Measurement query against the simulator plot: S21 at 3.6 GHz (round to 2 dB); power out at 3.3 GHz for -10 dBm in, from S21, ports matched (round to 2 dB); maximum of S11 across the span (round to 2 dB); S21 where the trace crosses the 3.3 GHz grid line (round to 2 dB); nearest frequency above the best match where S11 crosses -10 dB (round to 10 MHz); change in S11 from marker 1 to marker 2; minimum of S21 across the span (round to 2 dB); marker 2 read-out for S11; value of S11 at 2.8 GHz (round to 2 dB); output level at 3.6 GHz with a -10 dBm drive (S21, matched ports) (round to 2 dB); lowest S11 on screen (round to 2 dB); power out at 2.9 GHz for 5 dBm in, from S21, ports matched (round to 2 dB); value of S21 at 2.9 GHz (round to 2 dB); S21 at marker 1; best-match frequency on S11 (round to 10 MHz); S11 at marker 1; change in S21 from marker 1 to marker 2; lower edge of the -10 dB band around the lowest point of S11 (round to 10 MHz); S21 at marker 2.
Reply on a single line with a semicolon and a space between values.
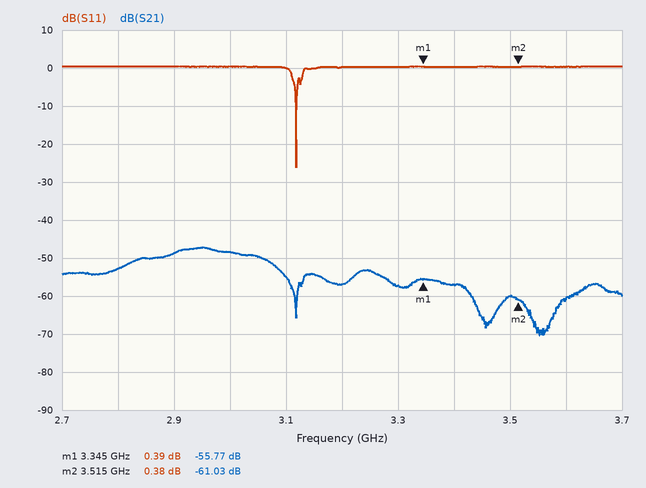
-60 dB; -68 dBm; 0 dB; -58 dB; 3.12 GHz; -0.01 dB; -70 dB; 0.38 dB; 0 dB; -70 dBm; -26 dB; -44 dBm; -48 dB; -55.77 dB; 3.12 GHz; 0.39 dB; -5.26 dB; 3.12 GHz; -61.03 dB
